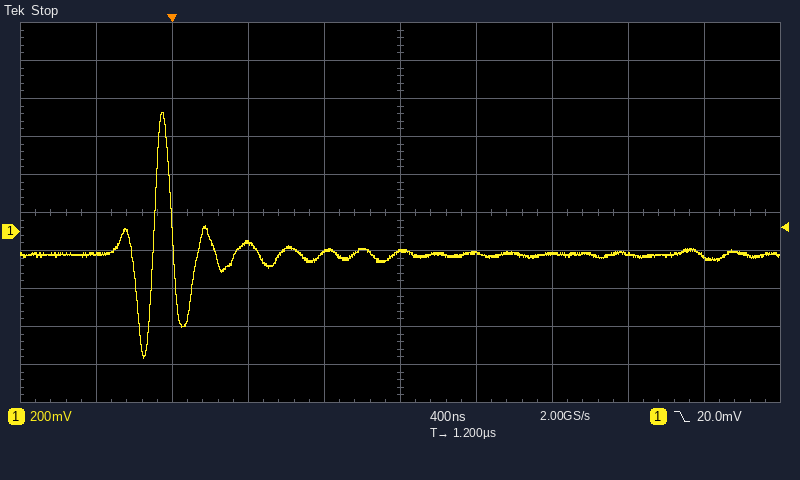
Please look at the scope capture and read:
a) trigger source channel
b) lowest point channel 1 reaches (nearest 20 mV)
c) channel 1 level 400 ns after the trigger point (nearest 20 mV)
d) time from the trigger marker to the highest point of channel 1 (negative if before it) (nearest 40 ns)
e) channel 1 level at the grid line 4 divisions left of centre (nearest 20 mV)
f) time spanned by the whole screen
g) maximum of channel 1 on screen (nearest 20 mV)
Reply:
channel 1
-660 mV
-60 mV
-40 ns
-120 mV
4 µs
620 mV
